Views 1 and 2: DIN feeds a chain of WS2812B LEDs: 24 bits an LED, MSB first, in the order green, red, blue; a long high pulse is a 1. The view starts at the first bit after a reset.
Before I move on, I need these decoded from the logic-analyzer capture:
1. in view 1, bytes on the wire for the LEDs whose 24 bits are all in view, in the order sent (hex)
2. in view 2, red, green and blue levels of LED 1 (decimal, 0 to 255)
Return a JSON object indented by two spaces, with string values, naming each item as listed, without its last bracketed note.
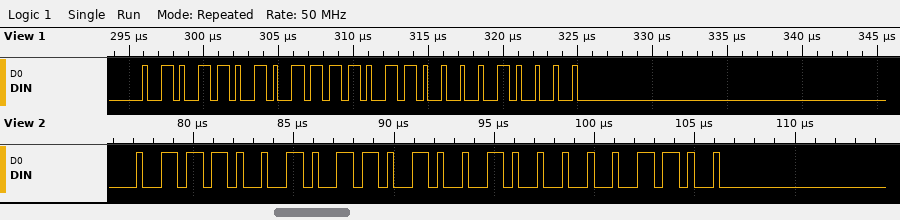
{
  "in view 1, bytes on the wire for the LEDs whose 24 bits are all in view, in the order sent": "5A F6 10",
  "in view 2, red, green and blue levels of LED 1": "210, 114, 12"
}
